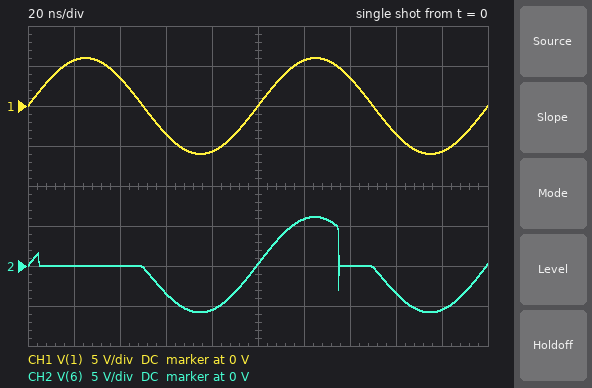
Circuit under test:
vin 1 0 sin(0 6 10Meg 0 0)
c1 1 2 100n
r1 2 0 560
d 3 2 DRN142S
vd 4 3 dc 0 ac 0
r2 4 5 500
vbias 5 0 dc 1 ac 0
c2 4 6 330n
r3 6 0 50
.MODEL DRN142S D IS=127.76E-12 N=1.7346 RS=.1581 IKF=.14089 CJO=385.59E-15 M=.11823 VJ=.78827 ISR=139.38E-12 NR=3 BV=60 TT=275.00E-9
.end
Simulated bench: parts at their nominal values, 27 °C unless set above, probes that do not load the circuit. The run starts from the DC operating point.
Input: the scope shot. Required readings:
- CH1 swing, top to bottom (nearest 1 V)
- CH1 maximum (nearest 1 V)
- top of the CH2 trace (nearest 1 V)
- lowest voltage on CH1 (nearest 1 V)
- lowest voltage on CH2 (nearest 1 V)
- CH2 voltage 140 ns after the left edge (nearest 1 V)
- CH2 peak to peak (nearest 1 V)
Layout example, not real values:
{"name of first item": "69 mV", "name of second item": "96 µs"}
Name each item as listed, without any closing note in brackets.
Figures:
{"CH1 swing, top to bottom": "12 V", "CH1 maximum": "6 V", "top of the CH2 trace": "6 V", "lowest voltage on CH1": "-6 V", "lowest voltage on CH2": "-6 V", "CH2 voltage 140 ns after the left edge": "0 V", "CH2 peak to peak": "12 V"}
